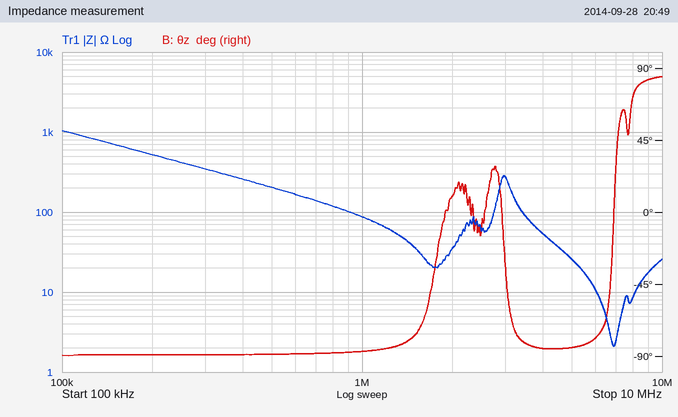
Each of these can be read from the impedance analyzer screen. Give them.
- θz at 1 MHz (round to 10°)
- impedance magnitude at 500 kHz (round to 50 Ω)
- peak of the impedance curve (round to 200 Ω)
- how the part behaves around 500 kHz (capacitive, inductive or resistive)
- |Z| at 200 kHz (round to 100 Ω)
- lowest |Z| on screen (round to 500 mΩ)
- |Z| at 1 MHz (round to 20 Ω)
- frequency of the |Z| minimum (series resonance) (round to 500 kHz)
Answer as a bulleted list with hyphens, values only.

- -90°
- 200 Ω
- 1.0 kΩ
- capacitive
- 500 Ω
- 2.0 Ω
- 80 Ω
- 7.0 MHz
